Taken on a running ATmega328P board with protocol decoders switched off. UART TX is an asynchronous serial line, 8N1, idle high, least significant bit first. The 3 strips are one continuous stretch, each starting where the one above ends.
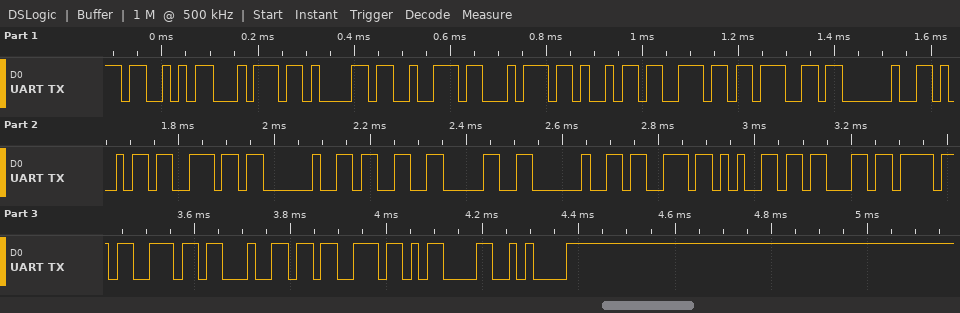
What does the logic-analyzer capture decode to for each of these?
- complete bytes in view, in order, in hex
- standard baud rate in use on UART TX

0x53 0x74 0x61 0x72 0x74 0x69 0x6E 0x67 0x20 0x69 0x6E 0x20 0x33 0x30 0x20 0x73 0x65 0x63 0x6F 0x6E 0x64 0x73 0x0D 0x0A
57600 baud
